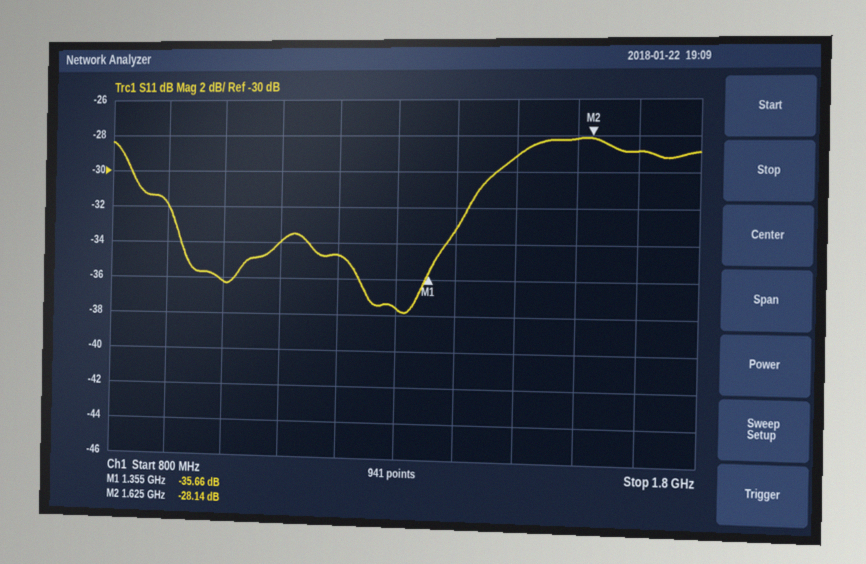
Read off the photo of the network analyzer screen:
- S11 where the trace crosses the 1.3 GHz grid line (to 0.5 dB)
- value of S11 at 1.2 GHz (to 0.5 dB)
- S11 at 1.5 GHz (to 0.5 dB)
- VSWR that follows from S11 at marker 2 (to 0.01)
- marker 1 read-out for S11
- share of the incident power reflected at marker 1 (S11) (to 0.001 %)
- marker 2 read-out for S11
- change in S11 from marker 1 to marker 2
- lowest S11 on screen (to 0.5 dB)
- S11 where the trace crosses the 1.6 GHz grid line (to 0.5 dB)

-37.5 dB
-34.5 dB
-29.0 dB
1.08
-35.66 dB
0.027 %
-28.14 dB
7.52 dB
-38.0 dB
-28.0 dB
